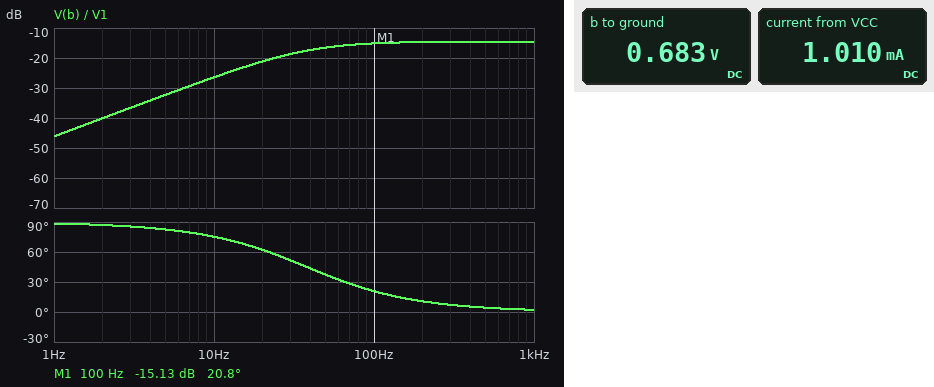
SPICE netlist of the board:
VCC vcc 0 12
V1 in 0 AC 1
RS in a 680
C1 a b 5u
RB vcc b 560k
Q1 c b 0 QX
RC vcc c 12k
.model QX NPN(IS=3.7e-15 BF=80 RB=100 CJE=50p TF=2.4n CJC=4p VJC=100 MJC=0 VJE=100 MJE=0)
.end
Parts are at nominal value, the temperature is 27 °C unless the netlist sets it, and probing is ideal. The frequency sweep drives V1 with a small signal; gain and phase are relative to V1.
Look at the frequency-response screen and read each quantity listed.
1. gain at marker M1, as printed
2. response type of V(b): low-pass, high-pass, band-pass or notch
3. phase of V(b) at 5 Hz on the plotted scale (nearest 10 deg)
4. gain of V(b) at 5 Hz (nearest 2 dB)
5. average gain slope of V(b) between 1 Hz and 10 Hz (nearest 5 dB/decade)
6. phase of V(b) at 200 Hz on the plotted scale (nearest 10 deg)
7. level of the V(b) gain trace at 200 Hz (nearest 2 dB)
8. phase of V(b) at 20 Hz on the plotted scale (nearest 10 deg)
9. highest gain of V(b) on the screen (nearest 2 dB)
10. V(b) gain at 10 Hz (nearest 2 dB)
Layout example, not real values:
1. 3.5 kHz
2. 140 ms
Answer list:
1. -15.13 dB
2. high-pass
3. 80 deg
4. -32 dB
5. 20 dB/decade
6. 10 deg
7. -14 dB
8. 60 deg
9. -14 dB
10. -26 dB
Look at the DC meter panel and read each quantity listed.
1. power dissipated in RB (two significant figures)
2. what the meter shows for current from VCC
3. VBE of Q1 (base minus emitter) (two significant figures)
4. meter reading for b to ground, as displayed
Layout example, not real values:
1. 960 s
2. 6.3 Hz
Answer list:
1. 230 µW
2. 1.010 mA
3. 680 mV
4. 0.683 V
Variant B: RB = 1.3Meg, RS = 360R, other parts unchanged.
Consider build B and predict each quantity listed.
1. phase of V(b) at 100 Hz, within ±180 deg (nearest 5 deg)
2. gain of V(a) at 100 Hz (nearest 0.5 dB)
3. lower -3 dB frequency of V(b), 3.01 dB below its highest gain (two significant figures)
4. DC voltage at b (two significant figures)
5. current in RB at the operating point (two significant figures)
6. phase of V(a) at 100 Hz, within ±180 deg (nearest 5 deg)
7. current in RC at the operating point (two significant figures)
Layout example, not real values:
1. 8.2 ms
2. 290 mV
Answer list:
1. 5 deg
2. -1.0 dB
3. 9.3 Hz
4. 670 mV
5. 8.7 µA
6. 0 deg
7. 700 µA
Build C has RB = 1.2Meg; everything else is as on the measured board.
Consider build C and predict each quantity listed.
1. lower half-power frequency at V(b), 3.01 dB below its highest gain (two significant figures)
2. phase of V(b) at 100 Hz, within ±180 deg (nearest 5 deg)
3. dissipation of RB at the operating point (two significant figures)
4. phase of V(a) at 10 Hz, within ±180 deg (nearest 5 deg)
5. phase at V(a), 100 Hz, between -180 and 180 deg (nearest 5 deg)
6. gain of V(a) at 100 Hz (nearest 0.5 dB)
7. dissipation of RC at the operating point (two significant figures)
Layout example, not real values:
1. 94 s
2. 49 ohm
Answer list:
1. 9.1 Hz
2. 5 deg
3. 110 µW
4. -5 deg
5. 0 deg
6. -2.0 dB
7. 6.8 mW
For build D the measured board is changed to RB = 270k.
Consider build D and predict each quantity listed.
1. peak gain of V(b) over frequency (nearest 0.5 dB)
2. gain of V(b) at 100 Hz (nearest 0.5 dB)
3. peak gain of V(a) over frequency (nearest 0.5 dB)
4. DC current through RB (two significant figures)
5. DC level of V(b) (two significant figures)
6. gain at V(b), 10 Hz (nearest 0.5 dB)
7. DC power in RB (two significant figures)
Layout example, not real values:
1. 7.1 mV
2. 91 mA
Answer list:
1. -15.0 dB
2. -15.5 dB
3. 0 dB
4. 42 µA
5. 690 mV
6. -27.0 dB
7. 470 µW
